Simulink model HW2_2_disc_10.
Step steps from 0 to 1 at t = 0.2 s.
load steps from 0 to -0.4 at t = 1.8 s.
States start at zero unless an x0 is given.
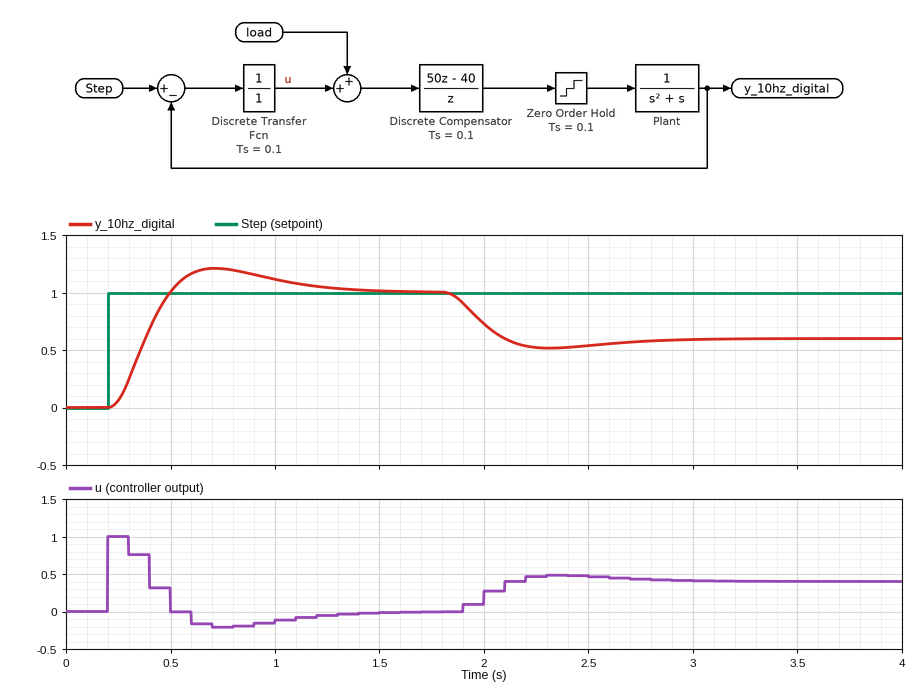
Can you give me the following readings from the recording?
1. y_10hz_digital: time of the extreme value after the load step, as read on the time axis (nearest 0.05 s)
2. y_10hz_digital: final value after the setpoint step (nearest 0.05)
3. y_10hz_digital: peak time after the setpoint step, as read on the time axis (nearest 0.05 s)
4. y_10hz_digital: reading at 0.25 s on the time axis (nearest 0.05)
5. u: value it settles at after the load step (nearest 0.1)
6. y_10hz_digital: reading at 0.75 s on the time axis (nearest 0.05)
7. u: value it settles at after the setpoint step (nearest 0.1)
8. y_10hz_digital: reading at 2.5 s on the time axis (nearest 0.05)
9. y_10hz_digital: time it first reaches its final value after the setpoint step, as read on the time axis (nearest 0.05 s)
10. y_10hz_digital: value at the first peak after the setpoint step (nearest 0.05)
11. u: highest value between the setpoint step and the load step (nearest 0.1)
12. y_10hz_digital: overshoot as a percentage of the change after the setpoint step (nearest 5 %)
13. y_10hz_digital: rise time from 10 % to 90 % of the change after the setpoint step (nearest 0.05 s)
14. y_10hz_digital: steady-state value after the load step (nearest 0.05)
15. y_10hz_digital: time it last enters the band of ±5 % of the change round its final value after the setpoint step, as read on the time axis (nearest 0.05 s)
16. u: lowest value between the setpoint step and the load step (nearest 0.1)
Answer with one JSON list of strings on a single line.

["2.30 s", "1.00", "0.70 s", "0.05", "0.4", "1.20", "0.0", "0.55", "0.50 s", "1.20", "1.0", "20 %", "0.20 s", "0.60", "1.20 s", "-0.2"]
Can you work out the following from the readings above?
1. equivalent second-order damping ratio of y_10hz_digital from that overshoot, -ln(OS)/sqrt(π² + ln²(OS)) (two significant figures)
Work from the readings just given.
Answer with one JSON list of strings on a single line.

["0.46"]
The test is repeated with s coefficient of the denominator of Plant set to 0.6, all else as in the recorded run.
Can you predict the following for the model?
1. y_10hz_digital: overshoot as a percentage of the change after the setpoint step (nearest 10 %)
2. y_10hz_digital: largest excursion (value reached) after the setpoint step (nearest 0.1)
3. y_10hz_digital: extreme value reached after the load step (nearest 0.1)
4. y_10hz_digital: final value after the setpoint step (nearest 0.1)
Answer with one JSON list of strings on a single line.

["30 %", "1.3", "0.5", "1.0"]
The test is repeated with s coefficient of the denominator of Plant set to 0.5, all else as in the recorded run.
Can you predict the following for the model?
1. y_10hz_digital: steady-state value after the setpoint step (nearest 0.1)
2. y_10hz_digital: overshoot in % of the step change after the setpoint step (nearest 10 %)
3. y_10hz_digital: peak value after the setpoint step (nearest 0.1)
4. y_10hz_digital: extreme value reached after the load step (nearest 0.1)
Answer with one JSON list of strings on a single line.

["1.0", "30 %", "1.3", "0.5"]
